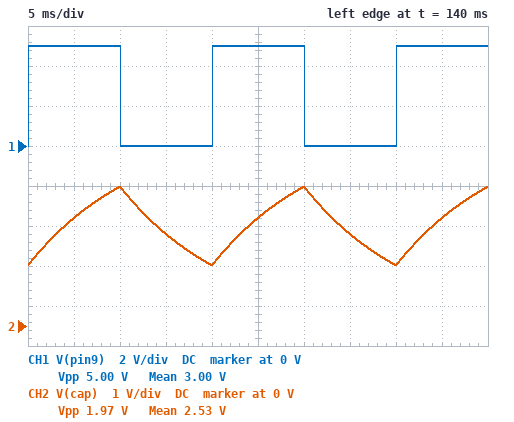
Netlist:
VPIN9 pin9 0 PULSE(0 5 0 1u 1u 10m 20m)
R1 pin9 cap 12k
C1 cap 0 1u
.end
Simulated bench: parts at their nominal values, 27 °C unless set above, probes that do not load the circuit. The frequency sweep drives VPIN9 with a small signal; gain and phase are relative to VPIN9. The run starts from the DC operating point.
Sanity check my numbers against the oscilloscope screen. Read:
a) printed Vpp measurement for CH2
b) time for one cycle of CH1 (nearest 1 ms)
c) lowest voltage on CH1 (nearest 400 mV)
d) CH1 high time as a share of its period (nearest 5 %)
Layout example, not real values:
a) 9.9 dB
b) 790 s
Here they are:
a) 1.97 V
b) 20 ms
c) 0 V
d) 50 %
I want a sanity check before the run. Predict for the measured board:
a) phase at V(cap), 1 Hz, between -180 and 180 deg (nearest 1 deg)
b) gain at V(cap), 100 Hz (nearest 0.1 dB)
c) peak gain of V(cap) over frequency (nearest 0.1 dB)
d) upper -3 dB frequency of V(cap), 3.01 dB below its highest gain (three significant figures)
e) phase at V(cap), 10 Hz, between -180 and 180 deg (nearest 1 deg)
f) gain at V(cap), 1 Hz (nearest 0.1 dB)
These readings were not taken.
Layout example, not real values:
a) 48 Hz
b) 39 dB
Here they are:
a) -4 deg
b) -17.6 dB
c) 0 dB
d) 13.3 Hz
e) -37 deg
f) 0 dB
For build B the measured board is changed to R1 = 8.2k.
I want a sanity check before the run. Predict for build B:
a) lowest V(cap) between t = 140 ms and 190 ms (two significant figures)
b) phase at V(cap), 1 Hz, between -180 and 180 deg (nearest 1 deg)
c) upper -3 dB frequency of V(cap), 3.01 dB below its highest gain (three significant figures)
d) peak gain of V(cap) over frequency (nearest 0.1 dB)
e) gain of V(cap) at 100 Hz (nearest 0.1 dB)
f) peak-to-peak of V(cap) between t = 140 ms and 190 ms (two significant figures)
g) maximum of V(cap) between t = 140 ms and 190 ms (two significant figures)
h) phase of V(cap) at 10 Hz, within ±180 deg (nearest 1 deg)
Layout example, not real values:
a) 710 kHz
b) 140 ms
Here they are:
a) 1.1 V
b) -3 deg
c) 19.4 Hz
d) 0 dB
e) -14.4 dB
f) 2.7 V
g) 3.9 V
h) -27 deg
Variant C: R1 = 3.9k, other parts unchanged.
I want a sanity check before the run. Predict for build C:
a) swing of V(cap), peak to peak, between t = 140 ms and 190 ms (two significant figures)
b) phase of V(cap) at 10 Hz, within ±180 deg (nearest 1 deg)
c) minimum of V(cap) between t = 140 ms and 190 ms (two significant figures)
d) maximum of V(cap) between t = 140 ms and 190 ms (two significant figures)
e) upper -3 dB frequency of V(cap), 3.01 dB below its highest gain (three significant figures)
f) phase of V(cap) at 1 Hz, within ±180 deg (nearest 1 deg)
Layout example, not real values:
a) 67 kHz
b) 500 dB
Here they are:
a) 4.3 V
b) -14 deg
c) 360 mV
d) 4.6 V
e) 40.8 Hz
f) -1 deg
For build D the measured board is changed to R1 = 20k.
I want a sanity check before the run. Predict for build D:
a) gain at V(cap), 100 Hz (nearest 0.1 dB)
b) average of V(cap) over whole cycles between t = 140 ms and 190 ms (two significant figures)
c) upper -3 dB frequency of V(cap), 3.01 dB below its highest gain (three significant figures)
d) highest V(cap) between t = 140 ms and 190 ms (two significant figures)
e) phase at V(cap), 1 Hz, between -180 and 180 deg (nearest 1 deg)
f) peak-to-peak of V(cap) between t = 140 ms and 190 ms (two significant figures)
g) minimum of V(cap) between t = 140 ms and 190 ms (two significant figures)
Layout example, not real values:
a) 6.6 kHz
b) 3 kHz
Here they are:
a) -22.0 dB
b) 2.5 V
c) 7.96 Hz
d) 3.1 V
e) -7 deg
f) 1.2 V
g) 1.9 V
